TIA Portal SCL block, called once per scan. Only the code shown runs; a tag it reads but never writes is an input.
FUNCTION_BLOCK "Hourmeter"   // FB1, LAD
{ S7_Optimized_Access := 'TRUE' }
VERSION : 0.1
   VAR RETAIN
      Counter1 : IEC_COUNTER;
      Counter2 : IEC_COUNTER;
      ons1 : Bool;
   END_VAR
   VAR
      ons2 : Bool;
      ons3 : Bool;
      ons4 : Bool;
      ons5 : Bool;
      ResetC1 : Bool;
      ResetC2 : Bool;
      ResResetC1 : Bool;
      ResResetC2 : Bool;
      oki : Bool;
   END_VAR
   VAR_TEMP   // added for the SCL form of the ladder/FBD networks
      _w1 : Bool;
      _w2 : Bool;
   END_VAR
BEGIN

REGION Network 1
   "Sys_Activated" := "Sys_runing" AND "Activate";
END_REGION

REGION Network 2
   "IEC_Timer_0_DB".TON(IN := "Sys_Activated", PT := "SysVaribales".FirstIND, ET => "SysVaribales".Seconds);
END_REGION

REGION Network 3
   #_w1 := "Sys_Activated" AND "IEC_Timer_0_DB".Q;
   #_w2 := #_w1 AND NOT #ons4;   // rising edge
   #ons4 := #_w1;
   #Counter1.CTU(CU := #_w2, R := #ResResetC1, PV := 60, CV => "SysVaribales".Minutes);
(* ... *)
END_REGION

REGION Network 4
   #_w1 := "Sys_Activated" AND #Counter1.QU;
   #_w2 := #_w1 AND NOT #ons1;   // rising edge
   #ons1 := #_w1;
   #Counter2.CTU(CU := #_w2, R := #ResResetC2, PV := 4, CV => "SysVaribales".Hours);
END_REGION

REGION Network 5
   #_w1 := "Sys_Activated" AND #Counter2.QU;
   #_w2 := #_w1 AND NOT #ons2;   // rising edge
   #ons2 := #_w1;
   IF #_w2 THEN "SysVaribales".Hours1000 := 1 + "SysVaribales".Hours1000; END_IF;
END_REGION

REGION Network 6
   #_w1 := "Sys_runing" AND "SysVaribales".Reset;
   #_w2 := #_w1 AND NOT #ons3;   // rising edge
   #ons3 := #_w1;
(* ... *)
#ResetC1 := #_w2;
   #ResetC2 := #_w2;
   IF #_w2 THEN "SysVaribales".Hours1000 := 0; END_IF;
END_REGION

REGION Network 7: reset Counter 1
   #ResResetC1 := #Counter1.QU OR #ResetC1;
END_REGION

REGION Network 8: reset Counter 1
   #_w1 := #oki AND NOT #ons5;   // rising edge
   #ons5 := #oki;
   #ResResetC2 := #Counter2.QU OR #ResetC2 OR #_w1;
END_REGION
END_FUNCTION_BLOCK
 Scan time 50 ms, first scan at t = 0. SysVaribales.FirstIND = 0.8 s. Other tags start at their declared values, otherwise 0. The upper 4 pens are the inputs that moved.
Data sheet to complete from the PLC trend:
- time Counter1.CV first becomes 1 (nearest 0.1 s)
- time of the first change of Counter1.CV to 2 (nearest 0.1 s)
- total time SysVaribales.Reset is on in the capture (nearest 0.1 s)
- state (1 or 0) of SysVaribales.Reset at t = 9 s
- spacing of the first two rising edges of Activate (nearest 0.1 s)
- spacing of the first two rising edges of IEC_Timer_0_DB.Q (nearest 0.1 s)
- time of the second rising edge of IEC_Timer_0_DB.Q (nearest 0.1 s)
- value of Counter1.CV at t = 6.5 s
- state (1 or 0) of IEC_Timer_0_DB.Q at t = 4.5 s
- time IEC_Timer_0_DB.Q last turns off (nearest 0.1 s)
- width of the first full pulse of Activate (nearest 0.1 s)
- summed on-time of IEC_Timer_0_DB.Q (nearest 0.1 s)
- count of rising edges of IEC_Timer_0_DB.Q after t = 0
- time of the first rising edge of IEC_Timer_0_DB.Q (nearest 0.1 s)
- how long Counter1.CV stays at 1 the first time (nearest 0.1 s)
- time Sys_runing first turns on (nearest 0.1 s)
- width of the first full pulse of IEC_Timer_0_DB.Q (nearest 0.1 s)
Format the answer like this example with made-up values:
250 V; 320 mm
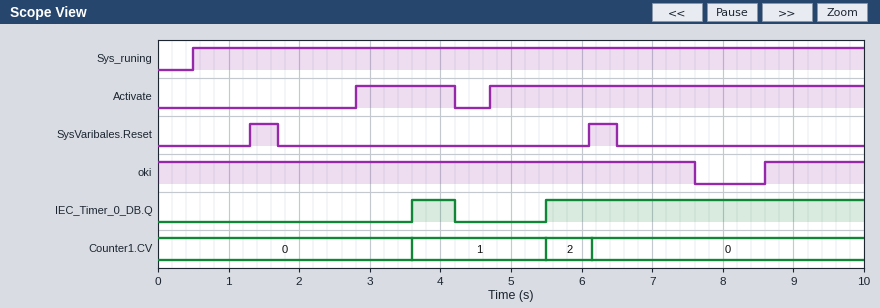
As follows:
3.6 s; 5.5 s; 0.8 s; 0; 1.9 s; 1.9 s; 5.5 s; 0; 0; 4.2 s; 1.4 s; 5.1 s; 2; 3.6 s; 1.9 s; 0.5 s; 0.6 s
